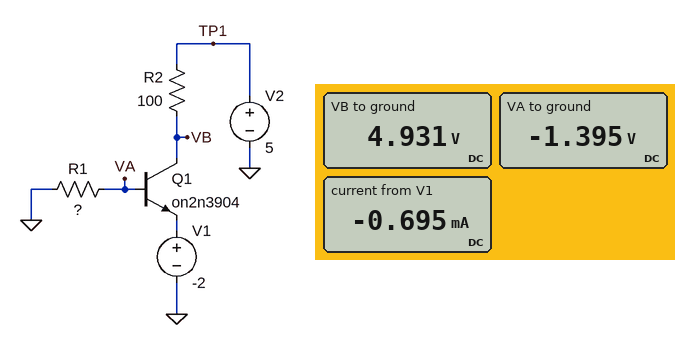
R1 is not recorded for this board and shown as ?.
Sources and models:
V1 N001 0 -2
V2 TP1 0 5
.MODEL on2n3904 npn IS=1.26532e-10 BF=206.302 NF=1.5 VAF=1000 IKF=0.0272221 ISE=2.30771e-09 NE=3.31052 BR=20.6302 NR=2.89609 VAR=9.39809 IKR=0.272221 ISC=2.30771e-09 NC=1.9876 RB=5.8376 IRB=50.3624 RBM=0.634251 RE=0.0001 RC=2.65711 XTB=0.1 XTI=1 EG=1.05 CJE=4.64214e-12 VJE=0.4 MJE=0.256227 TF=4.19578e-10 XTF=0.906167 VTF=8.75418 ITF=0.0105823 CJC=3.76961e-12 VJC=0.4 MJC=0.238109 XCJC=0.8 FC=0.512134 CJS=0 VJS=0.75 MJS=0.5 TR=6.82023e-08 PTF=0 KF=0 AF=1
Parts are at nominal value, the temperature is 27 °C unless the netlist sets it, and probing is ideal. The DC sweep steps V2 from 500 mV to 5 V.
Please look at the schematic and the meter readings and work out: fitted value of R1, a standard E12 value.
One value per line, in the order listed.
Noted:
220 kΩ
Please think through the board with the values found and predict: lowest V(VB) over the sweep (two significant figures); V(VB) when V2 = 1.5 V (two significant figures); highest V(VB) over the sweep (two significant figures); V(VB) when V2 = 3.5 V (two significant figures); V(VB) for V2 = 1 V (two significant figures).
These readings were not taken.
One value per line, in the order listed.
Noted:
430 mV
1.4 V
4.9 V
3.4 V
930 mV
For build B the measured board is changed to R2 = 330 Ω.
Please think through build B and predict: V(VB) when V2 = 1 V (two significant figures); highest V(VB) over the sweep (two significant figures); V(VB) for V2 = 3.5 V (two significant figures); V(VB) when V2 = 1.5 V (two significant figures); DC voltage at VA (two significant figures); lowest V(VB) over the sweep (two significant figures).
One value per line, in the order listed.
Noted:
770 mV
4.8 V
3.3 V
1.3 V
-1.4 V
270 mV
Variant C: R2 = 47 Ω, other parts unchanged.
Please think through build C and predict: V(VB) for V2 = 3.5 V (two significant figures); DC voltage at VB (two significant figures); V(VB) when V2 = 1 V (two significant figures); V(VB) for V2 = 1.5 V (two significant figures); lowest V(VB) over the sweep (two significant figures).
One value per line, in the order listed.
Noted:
3.5 V
5.0 V
970 mV
1.5 V
470 mV
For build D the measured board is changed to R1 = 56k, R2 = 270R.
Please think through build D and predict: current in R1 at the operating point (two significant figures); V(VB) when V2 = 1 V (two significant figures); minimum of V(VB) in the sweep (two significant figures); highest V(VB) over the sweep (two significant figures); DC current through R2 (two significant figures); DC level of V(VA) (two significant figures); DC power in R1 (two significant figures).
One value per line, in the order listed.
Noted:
24 µA
160 mV
-340 mV
4.2 V
3.1 mA
-1.3 V
32 µW
